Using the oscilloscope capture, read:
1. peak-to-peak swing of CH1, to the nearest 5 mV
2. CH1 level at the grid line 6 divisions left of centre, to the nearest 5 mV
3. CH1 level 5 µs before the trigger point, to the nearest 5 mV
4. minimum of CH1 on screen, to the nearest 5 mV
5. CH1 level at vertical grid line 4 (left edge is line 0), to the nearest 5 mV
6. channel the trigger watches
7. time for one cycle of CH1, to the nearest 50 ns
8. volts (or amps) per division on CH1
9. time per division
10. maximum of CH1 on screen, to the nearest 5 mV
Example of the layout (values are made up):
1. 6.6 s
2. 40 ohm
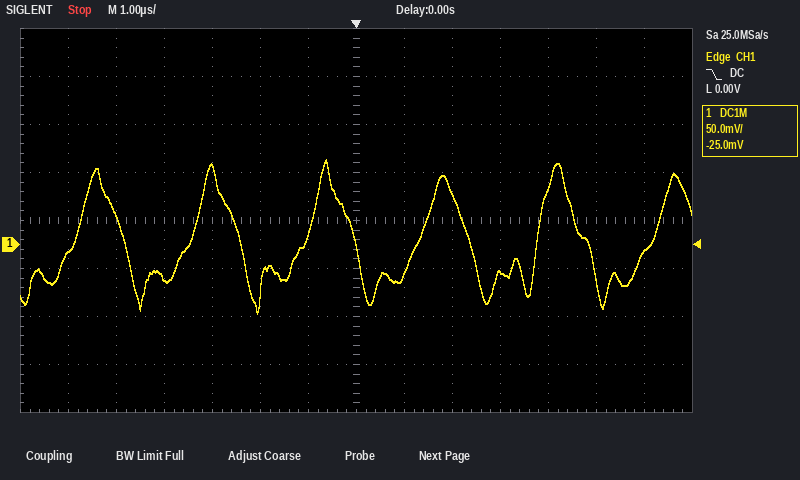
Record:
1. 160 mV
2. -10 mV
3. 30 mV
4. -70 mV
5. 80 mV
6. CH1
7. 2.40 µs
8. 50 mV
9. 1 µs
10. 90 mV
